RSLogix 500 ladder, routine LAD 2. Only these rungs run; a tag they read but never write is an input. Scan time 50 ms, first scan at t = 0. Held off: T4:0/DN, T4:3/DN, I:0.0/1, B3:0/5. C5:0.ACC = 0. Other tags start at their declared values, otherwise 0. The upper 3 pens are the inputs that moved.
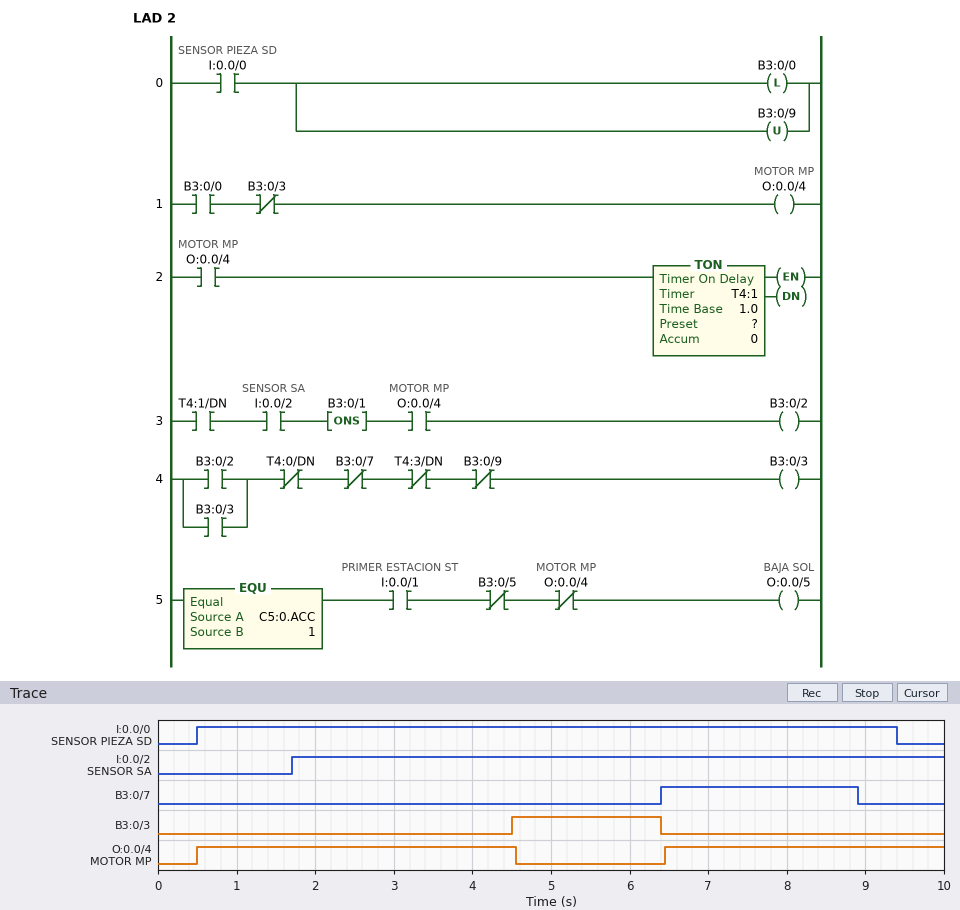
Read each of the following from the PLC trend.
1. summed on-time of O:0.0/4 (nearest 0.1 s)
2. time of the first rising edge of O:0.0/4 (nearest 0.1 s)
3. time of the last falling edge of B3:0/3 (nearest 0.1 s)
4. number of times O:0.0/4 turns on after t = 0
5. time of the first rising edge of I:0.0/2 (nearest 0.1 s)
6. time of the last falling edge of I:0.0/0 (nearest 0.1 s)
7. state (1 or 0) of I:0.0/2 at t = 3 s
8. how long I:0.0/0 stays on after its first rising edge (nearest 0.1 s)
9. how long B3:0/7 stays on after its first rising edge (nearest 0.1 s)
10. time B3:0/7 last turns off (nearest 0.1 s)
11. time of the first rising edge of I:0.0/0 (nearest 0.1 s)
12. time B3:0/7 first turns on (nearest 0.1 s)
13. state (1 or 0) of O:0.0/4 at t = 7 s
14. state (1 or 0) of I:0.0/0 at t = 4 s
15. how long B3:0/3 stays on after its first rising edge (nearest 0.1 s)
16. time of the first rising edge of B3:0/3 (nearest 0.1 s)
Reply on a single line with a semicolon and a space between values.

7.6 s; 0.5 s; 6.4 s; 2; 1.7 s; 9.4 s; 1; 8.9 s; 2.5 s; 8.9 s; 0.5 s; 6.4 s; 1; 1; 1.9 s; 4.5 s
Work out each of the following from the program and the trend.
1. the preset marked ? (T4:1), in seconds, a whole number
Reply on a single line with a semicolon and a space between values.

4 s
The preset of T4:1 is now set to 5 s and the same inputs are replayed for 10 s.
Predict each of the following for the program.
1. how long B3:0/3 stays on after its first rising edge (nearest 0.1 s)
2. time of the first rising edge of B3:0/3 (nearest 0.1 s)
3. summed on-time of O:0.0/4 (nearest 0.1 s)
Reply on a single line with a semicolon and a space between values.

0.9 s; 5.5 s; 8.6 s
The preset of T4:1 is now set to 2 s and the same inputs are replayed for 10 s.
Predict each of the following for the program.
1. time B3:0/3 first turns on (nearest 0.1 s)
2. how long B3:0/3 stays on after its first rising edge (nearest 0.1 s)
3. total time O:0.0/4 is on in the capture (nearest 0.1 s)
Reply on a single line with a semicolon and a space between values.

2.5 s; 3.9 s; 5.6 s
